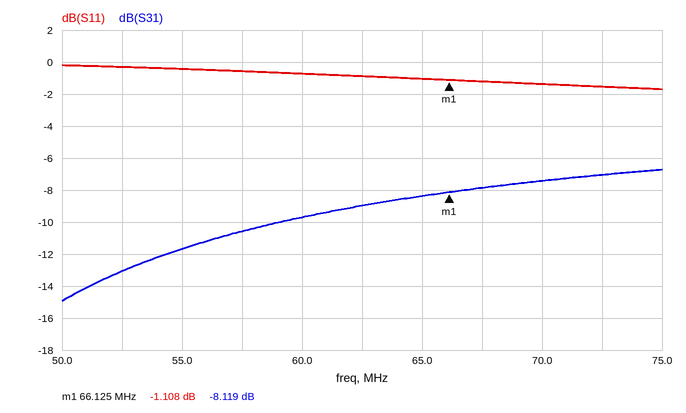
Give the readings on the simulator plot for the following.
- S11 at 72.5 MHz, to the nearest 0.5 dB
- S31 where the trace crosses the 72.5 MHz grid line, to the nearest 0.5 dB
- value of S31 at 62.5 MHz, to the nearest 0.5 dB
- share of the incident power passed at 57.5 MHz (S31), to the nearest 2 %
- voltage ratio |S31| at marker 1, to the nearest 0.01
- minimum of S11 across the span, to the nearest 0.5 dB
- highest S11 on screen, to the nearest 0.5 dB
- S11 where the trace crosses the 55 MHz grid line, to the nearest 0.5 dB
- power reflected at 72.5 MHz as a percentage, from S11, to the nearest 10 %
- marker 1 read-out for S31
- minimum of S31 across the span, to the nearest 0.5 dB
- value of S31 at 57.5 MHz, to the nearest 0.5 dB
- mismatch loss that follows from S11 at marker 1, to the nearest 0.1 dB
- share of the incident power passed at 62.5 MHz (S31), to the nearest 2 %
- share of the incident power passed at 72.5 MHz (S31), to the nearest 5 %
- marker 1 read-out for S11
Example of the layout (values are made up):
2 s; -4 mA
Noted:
-1.5 dB; -7.0 dB; -9.0 dB; 8 %; 0.39; -1.5 dB; 0.0 dB; -0.5 dB; 70 %; -8.119 dB; -15.0 dB; -10.5 dB; 6.5 dB; 12 %; 20 %; -1.108 dB
